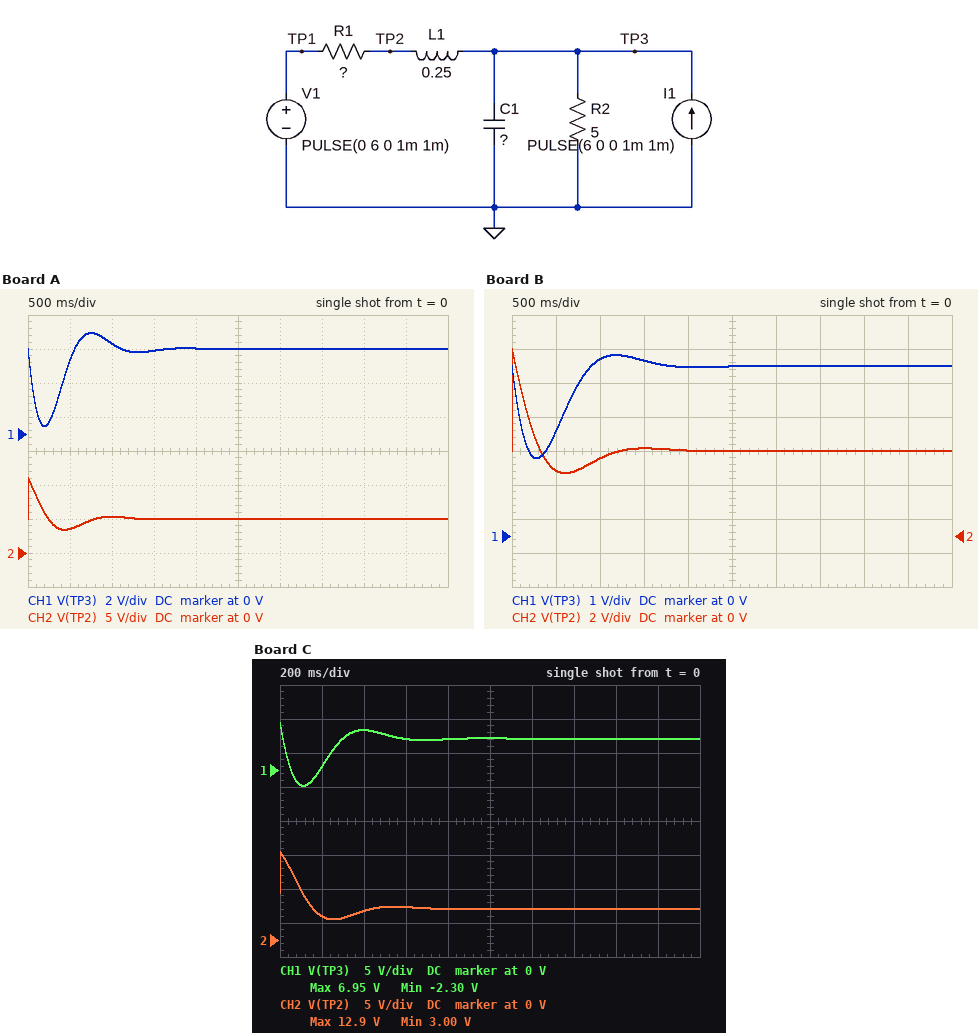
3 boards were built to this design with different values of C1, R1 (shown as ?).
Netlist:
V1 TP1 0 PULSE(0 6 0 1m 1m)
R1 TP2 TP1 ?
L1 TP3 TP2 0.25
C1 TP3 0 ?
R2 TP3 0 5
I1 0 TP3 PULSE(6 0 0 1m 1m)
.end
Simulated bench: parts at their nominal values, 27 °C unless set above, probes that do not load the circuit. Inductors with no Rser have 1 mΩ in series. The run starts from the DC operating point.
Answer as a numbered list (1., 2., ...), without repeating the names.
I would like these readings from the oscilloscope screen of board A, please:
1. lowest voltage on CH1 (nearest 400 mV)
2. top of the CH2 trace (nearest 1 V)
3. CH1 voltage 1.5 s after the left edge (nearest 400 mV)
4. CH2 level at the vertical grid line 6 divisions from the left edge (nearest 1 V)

1. 400 mV
2. 11 V
3. 4.8 V
4. 5 V
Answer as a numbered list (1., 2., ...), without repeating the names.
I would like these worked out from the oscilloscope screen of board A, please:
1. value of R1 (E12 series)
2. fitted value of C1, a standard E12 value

1. 1 Ω
2. 120 mF
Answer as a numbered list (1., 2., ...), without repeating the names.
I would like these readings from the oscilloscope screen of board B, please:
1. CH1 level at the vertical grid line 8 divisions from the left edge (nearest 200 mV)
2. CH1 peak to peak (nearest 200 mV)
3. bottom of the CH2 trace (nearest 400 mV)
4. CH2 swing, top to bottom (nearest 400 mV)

1. 5.0 V
2. 3.0 V
3. 3.6 V
4. 7.2 V
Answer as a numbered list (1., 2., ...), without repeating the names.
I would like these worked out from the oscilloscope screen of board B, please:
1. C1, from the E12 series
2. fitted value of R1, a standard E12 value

1. 270 mF
2. 1 Ω
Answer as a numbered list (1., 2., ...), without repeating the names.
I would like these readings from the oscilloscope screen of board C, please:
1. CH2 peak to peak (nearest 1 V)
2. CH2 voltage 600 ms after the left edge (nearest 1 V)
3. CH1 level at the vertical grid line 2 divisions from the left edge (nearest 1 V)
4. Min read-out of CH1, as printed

1. 10 V
2. 5 V
3. 6 V
4. -2.30 V
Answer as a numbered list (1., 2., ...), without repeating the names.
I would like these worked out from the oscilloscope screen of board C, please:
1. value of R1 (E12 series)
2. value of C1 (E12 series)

1. 1.5 Ω
2. 33 mF
